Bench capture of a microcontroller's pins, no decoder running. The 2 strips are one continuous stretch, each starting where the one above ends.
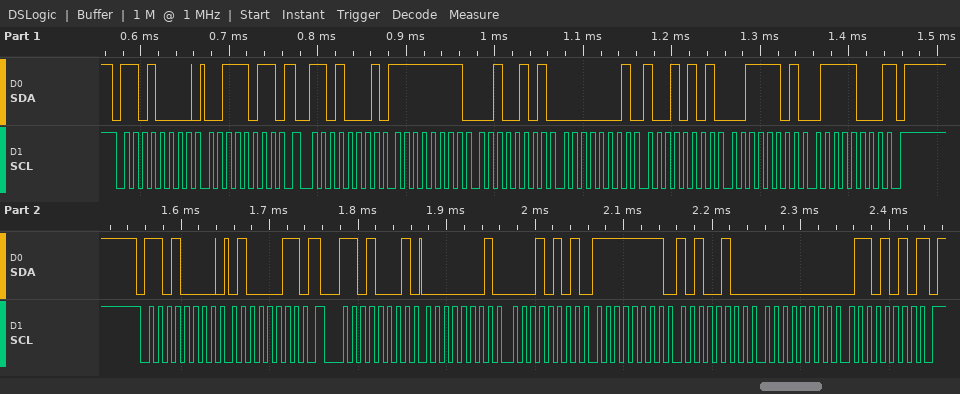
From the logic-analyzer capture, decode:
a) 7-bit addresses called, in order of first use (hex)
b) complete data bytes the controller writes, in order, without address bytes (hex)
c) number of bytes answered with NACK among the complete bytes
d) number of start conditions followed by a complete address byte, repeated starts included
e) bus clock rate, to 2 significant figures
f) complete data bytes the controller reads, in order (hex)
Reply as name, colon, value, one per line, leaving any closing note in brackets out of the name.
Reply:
7-bit addresses called, in order of first use: 0x68
complete data bytes the controller writes, in order, without address bytes: 3B 43
number of bytes answered with NACK among the complete bytes: 2
number of start conditions followed by a complete address byte, repeated starts included: 4
bus clock rate, to 2 significant figures: 100 kHz
complete data bytes the controller reads, in order: FF 25 01 95 3D 78 01 15 FF A4 00 6A
